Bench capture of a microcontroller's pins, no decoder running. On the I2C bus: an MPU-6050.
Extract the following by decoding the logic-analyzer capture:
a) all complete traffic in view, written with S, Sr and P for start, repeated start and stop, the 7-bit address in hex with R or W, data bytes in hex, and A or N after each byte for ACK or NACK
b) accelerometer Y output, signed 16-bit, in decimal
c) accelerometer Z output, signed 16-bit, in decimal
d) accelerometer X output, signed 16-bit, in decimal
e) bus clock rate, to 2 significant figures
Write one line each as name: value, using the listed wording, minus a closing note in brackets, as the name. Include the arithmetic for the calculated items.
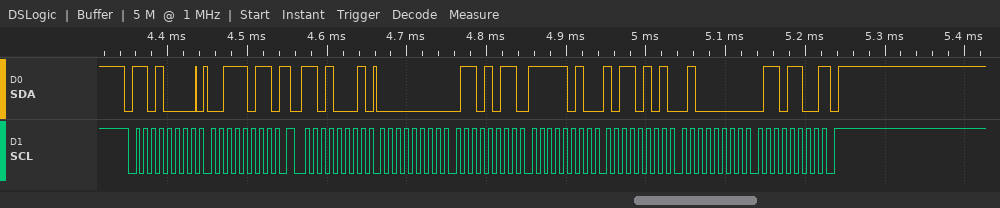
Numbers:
all complete traffic in view, written with S, Sr and P for start, repeated start and stop, the 7-bit address in hex with R or W, data bytes in hex, and A or N after each byte for ACK or NACK: S 68W A 3B A Sr 68R A 00 A 6B A FA A B5 A 40 A 6C N P
accelerometer Y output, signed 16-bit, in decimal: 0xFAB5 = -1355
accelerometer Z output, signed 16-bit, in decimal: 0x406C = 16492
accelerometer X output, signed 16-bit, in decimal: 0x006B = 107
bus clock rate, to 2 significant figures: 100 kHz
